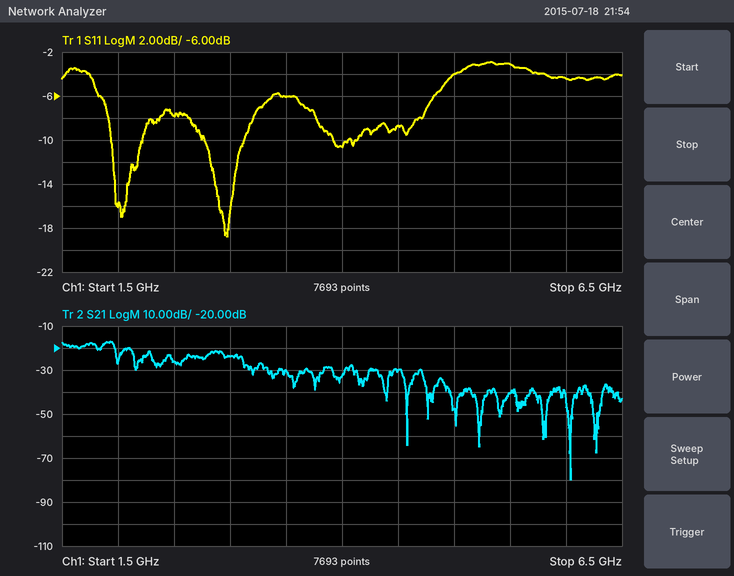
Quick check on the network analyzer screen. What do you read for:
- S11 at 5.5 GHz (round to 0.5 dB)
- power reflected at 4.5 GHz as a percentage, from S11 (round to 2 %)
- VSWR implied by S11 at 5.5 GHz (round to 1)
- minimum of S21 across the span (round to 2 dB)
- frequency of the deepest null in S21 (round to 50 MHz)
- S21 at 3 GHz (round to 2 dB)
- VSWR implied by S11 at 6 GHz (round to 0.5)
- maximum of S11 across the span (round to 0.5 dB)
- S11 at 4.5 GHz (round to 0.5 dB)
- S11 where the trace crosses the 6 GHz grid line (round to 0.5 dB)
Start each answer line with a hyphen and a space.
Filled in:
- -3.0 dB
- 14 %
- 6
- -80 dB
- 6.05 GHz
- -24 dB
- 4.0
- -3.0 dB
- -8.5 dB
- -4.5 dB
